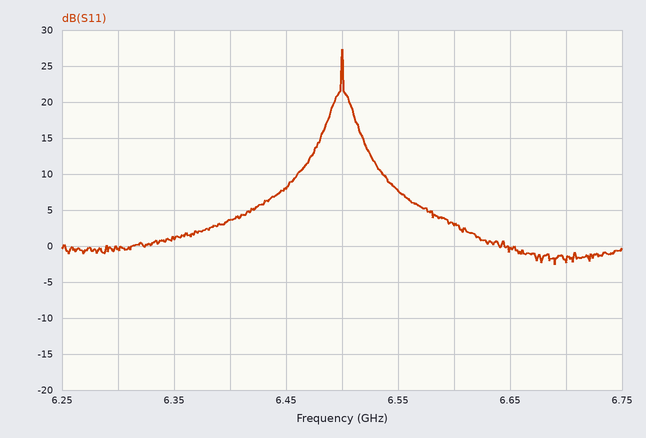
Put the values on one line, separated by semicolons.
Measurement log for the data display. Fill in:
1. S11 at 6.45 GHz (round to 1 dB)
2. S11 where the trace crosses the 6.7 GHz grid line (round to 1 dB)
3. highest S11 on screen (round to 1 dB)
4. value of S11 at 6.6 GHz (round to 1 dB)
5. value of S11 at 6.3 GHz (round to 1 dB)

8 dB; -2 dB; 27 dB; 3 dB; 0 dB
